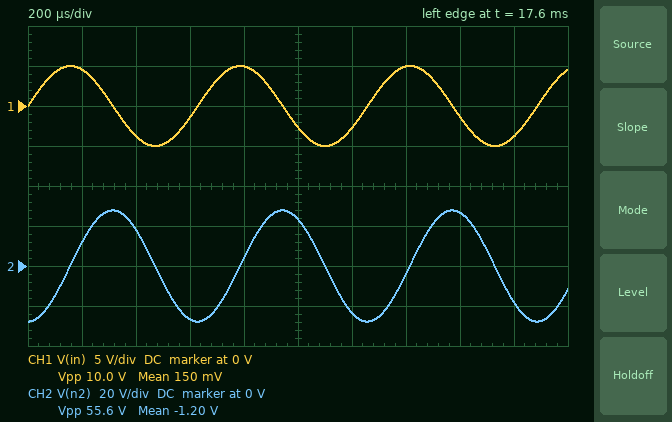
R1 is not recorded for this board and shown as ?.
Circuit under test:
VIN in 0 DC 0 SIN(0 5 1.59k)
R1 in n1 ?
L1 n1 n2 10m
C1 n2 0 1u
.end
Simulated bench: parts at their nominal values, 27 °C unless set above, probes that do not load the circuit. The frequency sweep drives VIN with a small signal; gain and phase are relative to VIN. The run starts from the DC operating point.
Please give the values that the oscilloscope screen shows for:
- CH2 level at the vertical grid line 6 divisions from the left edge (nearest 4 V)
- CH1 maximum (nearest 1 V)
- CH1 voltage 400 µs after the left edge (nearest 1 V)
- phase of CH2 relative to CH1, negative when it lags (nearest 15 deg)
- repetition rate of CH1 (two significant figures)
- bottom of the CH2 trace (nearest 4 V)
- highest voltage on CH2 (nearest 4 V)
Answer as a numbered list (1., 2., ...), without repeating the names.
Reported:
1. -24 V
2. 5 V
3. -4 V
4. -90 deg
5. 1.6 kHz
6. -28 V
7. 28 V
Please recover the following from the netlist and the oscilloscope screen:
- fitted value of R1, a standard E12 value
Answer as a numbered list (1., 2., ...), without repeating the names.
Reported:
1. 18 Ω
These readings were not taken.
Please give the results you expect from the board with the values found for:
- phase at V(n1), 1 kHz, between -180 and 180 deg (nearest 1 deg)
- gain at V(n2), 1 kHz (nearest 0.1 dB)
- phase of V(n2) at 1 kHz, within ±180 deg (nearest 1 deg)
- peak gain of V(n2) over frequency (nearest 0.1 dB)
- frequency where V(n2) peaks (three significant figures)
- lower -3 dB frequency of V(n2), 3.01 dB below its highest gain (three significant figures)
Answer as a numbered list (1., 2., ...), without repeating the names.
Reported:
1. -11 deg
2. 4.2 dB
3. -11 deg
4. 14.9 dB
5. 1.58 kHz
6. 1.43 kHz
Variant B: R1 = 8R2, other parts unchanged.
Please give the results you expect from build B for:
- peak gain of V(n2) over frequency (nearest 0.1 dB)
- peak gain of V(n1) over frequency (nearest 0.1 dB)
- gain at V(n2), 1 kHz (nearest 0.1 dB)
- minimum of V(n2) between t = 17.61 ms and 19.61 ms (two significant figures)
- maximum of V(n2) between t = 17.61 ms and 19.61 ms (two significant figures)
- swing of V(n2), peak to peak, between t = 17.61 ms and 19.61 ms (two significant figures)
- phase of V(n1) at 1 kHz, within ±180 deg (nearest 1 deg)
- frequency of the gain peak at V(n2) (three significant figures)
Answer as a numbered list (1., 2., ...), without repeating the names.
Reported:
1. 21.7 dB
2. 0 dB
3. 4.3 dB
4. -61 V
5. 61 V
6. 120 V
7. -5 deg
8. 1.59 kHz
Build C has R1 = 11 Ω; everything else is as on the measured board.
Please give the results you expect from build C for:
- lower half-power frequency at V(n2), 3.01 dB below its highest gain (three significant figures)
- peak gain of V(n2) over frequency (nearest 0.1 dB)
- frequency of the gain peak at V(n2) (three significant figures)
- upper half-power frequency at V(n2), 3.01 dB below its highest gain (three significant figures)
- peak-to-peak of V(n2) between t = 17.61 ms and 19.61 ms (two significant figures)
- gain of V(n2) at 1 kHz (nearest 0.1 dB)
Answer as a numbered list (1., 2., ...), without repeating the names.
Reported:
1. 1.50 kHz
2. 19.2 dB
3. 1.59 kHz
4. 1.67 kHz
5. 91 V
6. 4.3 dB
